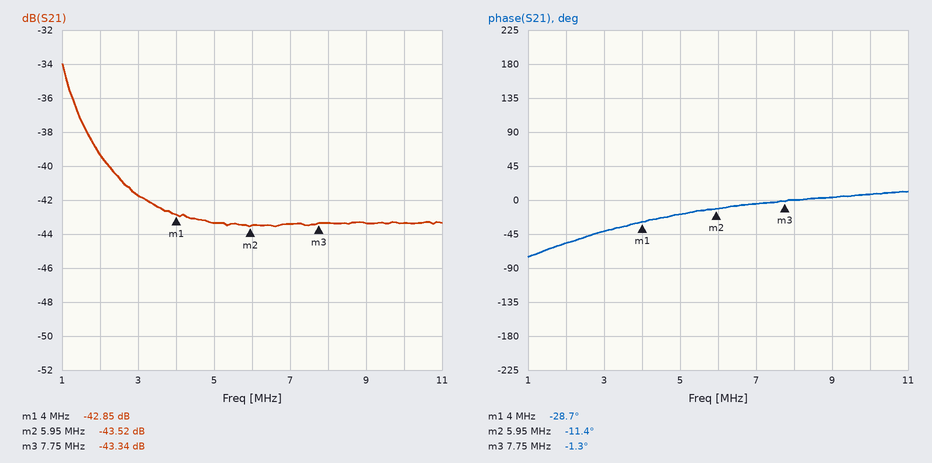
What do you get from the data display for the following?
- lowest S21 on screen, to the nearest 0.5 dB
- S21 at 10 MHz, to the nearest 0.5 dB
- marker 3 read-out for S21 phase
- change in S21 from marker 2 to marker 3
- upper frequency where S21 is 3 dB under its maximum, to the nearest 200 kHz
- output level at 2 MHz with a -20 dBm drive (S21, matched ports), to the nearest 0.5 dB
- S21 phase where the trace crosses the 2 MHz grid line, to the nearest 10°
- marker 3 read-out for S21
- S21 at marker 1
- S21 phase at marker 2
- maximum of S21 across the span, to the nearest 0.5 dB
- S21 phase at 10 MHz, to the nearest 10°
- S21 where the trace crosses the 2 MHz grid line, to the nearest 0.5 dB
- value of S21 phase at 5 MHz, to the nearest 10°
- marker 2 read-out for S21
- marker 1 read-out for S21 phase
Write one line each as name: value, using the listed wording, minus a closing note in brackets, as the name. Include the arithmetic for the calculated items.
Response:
lowest S21 on screen, to the nearest 0.5 dB: -43.5 dB
S21 at 10 MHz, to the nearest 0.5 dB: -43.5 dB
marker 3 read-out for S21 phase: -1.3°
change in S21 from marker 2 to marker 3: -43.34 − (-43.52) = 0.18 dB
upper frequency where S21 is 3 dB under its maximum, to the nearest 200 kHz: 1.4 MHz
output level at 2 MHz with a -20 dBm drive (S21, matched ports), to the nearest 0.5 dB: -20 dBm + (-39.5 dB) = -59.5 dBm
S21 phase where the trace crosses the 2 MHz grid line, to the nearest 10°: -60°
marker 3 read-out for S21: -43.34 dB
S21 at marker 1: -42.85 dB
S21 phase at marker 2: -11.4°
maximum of S21 across the span, to the nearest 0.5 dB: -34.0 dB
S21 phase at 10 MHz, to the nearest 10°: 10°
S21 where the trace crosses the 2 MHz grid line, to the nearest 0.5 dB: -39.5 dB
value of S21 phase at 5 MHz, to the nearest 10°: -20°
marker 2 read-out for S21: -43.52 dB
marker 1 read-out for S21 phase: -28.7°
